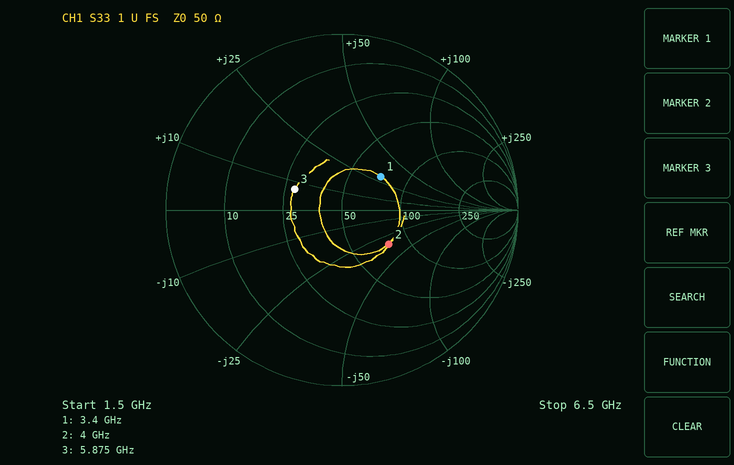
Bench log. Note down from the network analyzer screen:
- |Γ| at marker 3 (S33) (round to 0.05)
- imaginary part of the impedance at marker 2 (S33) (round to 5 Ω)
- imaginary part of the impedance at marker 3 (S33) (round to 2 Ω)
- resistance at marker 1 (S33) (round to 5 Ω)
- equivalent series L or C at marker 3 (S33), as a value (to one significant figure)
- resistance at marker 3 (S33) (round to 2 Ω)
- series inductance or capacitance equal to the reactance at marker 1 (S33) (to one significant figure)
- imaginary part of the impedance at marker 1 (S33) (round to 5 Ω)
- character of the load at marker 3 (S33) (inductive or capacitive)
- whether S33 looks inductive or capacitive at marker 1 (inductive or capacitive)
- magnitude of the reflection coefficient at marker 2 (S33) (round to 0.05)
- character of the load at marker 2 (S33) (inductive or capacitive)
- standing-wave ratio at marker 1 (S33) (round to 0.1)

0.30
-35 Ω
+8 Ω
70 Ω
200 pH
28 Ω
1 nH
+30 Ω
inductive
inductive
0.35
capacitive
1.8
